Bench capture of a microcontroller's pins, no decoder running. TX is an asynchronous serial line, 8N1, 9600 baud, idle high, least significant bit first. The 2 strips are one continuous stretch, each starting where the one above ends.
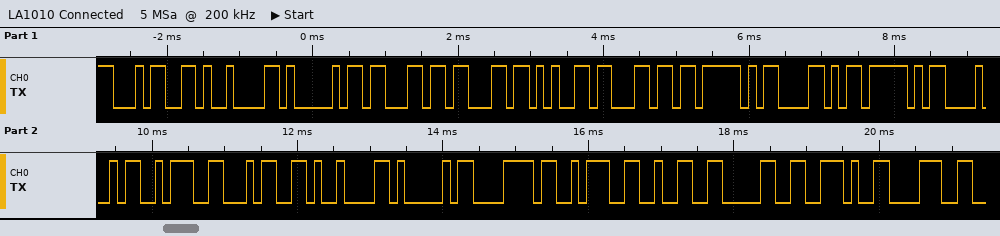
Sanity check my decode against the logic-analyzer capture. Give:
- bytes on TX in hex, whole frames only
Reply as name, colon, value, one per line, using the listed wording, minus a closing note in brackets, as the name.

bytes on TX in hex, whole frames only: 34 09 41 63 63 65 6C 5F 58 5F 48 3A 34 09 41 78 3A 32 30 2E 38
